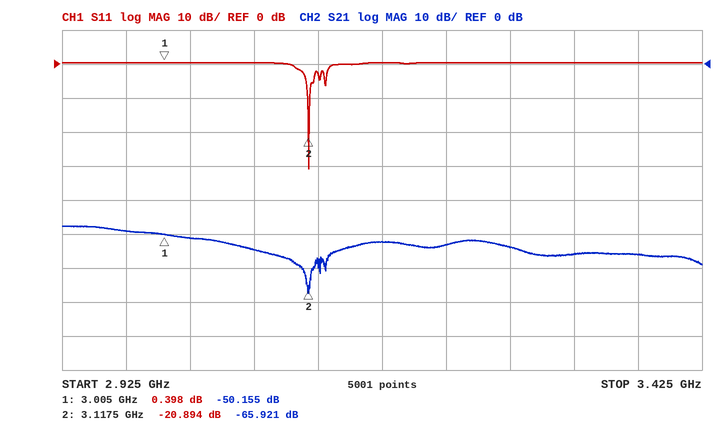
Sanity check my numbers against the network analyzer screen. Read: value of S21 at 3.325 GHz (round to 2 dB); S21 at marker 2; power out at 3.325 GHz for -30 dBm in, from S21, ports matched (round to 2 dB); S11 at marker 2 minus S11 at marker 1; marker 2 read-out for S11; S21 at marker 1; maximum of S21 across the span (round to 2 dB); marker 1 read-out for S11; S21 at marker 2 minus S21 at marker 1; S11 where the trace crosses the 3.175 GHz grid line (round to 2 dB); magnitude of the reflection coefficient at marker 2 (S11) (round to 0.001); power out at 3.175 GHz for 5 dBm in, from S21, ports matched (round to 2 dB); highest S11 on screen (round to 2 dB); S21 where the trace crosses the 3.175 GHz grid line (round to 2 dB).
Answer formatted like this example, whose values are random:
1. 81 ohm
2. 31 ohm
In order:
1. -56 dB
2. -65.921 dB
3. -86 dBm
4. -21.292 dB
5. -20.894 dB
6. -50.155 dB
7. -48 dB
8. 0.398 dB
9. -15.766 dB
10. 0 dB
11. 0.090
12. -48 dBm
13. 0 dB
14. -52 dB
